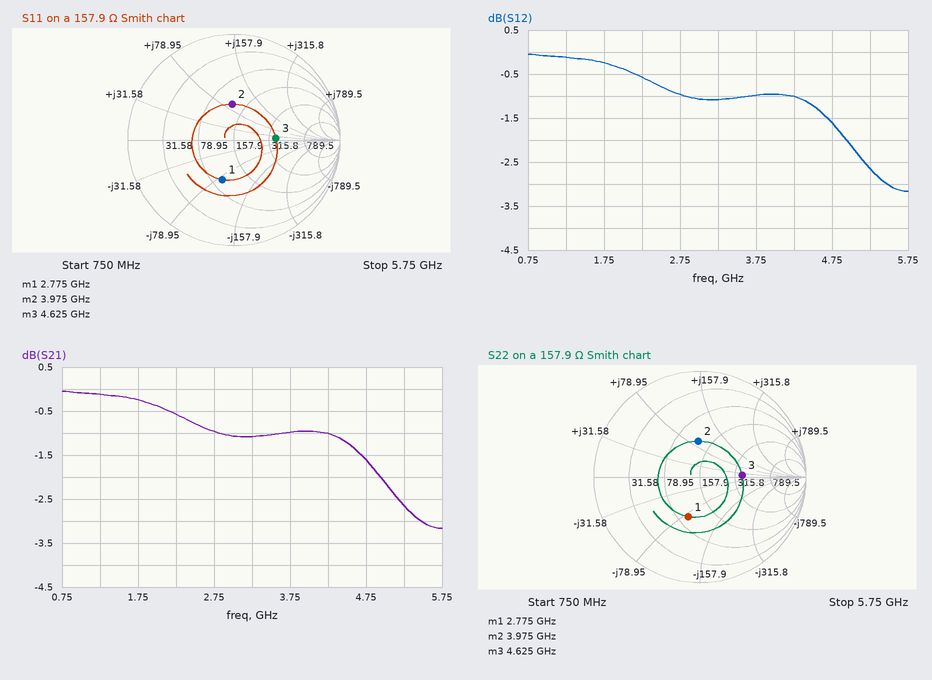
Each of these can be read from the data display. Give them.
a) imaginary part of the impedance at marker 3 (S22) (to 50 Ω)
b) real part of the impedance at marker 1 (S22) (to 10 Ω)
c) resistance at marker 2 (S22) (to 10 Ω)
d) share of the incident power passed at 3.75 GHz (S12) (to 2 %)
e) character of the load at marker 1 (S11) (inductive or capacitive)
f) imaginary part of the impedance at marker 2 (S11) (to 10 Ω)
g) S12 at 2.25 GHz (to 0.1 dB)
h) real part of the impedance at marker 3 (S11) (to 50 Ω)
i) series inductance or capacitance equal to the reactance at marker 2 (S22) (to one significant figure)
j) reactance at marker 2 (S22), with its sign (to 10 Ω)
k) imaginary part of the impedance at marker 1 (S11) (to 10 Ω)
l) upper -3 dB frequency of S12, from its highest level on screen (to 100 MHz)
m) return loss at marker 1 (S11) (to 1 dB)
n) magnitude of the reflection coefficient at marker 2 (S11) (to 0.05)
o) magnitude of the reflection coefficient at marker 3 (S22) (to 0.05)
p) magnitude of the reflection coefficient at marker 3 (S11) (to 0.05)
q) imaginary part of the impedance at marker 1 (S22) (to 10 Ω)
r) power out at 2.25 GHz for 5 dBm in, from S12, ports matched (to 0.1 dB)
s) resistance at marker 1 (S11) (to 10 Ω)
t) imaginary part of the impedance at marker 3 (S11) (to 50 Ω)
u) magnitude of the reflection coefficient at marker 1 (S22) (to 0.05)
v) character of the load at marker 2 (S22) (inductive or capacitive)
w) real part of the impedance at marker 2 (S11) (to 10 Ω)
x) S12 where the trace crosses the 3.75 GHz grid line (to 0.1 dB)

0 Ω
100 Ω
120 Ω
80 %
capacitive
+90 Ω
-0.6 dB
350 Ω
4 nH
+90 Ω
-90 Ω
5.5 GHz
8 dB
0.35
0.40
0.40
-90 Ω
4.4 dBm
100 Ω
0 Ω
0.40
inductive
120 Ω
-1.0 dB
